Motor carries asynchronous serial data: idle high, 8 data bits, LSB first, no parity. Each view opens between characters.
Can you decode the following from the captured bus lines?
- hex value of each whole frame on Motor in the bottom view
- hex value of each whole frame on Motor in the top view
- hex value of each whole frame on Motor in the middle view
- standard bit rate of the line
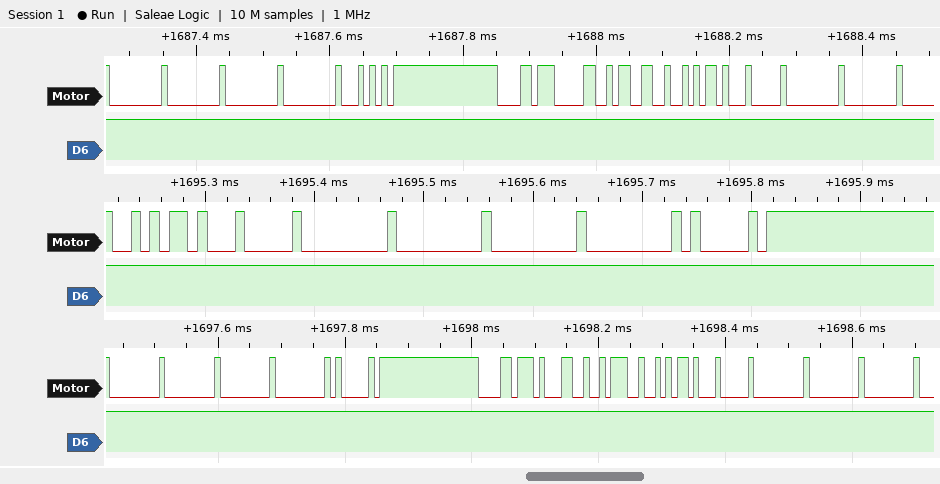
00, 00, 00, 00, 41, D8, 31, 3A, 6A, 04, 00, 00, 00
00, 00, 00, 00, 54, D8, 30, 33, 6A, 04, 00, 00
6A, 04, 00, 00, 00, 00, 41
115200 baud
